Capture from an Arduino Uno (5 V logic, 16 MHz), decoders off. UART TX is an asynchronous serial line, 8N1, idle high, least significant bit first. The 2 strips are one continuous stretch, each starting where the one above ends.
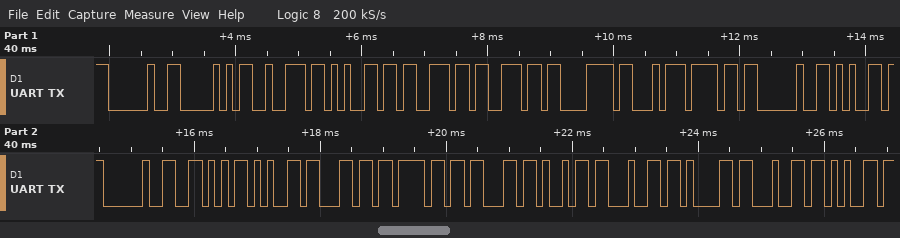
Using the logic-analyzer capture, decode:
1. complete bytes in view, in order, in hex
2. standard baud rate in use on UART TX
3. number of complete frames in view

20 50 72 65 73 73 C3 A3 6F 20 65 20 56 65 6C 6F 63 69 64 61 64 65
9600 baud
22
